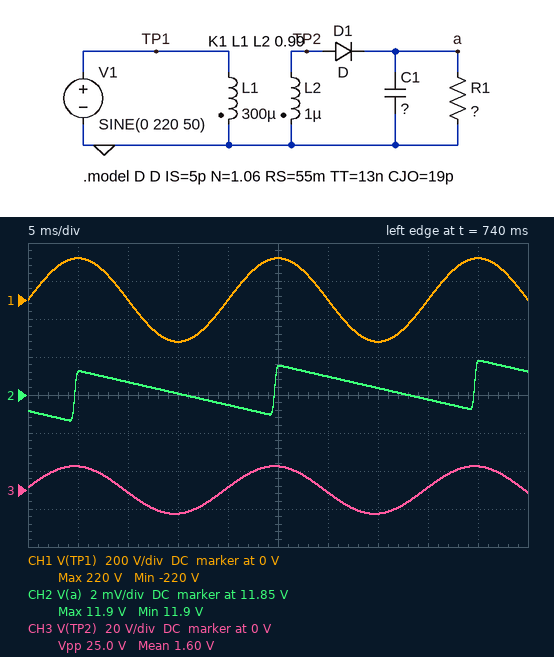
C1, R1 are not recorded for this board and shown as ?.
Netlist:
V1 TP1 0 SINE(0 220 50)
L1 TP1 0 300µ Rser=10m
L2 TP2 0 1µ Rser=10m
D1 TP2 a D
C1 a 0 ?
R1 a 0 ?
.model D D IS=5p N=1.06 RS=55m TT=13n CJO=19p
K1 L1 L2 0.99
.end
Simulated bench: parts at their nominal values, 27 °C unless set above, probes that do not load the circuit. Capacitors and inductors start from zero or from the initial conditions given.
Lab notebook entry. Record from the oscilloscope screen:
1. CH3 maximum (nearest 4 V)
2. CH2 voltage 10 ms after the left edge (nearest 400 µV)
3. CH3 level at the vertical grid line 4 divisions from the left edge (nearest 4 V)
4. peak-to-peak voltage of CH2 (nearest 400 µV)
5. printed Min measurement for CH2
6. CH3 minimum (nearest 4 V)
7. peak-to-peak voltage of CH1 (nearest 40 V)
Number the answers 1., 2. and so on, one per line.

1. 12 V
2. 11.8548 V
3. 0 V
4. 3.2 mV
5. 11.9 V
6. -12 V
7. 440 V
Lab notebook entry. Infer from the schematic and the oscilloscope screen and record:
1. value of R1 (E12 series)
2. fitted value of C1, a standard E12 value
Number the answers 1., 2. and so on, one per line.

1. 8.2 kΩ
2. 12 mF
